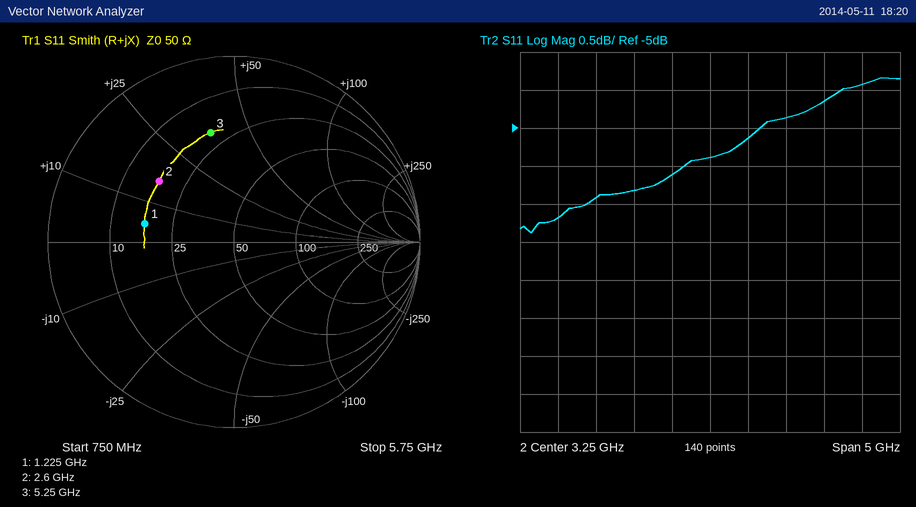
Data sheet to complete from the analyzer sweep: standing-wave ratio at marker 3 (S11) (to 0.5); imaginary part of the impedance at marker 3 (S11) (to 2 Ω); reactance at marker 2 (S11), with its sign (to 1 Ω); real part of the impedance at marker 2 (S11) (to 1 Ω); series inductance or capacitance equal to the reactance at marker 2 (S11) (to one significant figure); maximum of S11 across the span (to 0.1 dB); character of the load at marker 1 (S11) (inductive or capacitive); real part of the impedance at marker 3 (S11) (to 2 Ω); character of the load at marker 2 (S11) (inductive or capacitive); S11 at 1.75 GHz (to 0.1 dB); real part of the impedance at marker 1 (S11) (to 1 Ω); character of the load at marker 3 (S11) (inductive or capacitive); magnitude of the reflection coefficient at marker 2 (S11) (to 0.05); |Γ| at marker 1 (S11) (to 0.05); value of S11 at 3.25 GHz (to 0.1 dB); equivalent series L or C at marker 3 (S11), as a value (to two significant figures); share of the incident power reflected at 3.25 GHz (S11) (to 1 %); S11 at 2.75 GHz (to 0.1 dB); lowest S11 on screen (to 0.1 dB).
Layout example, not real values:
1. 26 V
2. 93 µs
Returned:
1. 4.0
2. +36 Ω
3. +16 Ω
4. 18 Ω
5. 1.0 nH
6. -4.3 dB
7. inductive
8. 20 Ω
9. inductive
10. -5.9 dB
11. 17 Ω
12. inductive
13. 0.50
14. 0.50
15. -5.4 dB
16. 1.1 nH
17. 29 %
18. -5.6 dB
19. -6.4 dB
